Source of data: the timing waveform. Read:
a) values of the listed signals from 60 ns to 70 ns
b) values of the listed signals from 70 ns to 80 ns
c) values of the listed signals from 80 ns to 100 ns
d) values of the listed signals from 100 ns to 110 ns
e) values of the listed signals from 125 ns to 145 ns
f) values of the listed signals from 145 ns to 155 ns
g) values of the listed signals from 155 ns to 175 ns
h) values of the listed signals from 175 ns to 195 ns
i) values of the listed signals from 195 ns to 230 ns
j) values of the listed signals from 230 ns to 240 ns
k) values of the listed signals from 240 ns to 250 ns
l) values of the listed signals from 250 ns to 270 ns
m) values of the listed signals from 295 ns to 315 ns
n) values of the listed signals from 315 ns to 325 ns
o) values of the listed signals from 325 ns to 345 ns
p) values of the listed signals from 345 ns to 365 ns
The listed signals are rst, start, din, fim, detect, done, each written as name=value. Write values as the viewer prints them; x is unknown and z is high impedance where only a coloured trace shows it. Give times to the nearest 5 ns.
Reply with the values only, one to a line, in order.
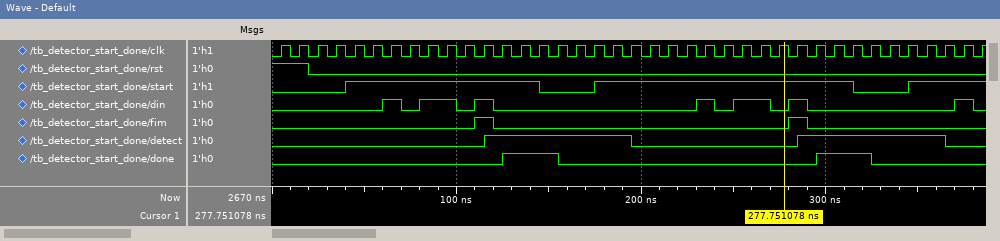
rst=0, start=1, din=1, fim=0, detect=0, done=0
rst=0, start=1, din=0, fim=0, detect=0, done=0
rst=0, start=1, din=1, fim=0, detect=0, done=0
rst=0, start=1, din=0, fim=0, detect=0, done=0
rst=0, start=1, din=0, fim=0, detect=1, done=1
rst=0, start=0, din=0, fim=0, detect=1, done=1
rst=0, start=0, din=0, fim=0, detect=1, done=0
rst=0, start=1, din=0, fim=0, detect=1, done=0
rst=0, start=1, din=0, fim=0, detect=0, done=0
rst=0, start=1, din=1, fim=0, detect=0, done=0
rst=0, start=1, din=0, fim=0, detect=0, done=0
rst=0, start=1, din=1, fim=0, detect=0, done=0
rst=0, start=1, din=0, fim=0, detect=1, done=1
rst=0, start=0, din=0, fim=0, detect=1, done=1
rst=0, start=0, din=0, fim=0, detect=1, done=0
rst=0, start=1, din=0, fim=0, detect=1, done=0
